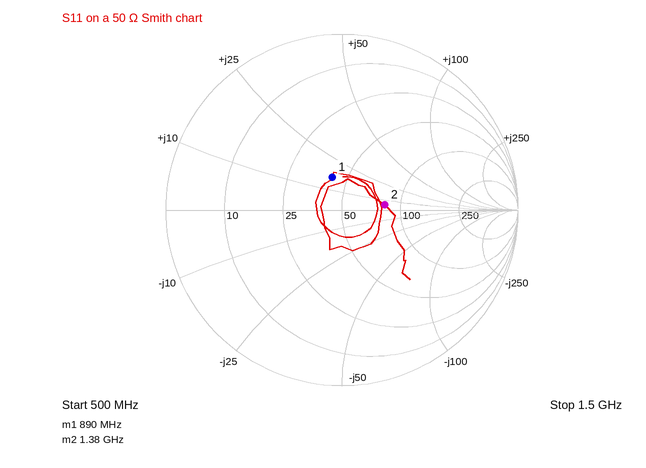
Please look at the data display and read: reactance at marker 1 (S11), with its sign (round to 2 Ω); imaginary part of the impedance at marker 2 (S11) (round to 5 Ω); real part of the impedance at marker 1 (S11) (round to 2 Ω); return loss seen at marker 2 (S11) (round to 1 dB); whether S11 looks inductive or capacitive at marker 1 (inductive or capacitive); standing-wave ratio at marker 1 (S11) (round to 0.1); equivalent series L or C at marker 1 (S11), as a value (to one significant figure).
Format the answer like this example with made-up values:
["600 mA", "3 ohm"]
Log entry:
["+16 Ω", "+5 Ω", "42 Ω", "12 dB", "inductive", "1.5", "3 nH"]
